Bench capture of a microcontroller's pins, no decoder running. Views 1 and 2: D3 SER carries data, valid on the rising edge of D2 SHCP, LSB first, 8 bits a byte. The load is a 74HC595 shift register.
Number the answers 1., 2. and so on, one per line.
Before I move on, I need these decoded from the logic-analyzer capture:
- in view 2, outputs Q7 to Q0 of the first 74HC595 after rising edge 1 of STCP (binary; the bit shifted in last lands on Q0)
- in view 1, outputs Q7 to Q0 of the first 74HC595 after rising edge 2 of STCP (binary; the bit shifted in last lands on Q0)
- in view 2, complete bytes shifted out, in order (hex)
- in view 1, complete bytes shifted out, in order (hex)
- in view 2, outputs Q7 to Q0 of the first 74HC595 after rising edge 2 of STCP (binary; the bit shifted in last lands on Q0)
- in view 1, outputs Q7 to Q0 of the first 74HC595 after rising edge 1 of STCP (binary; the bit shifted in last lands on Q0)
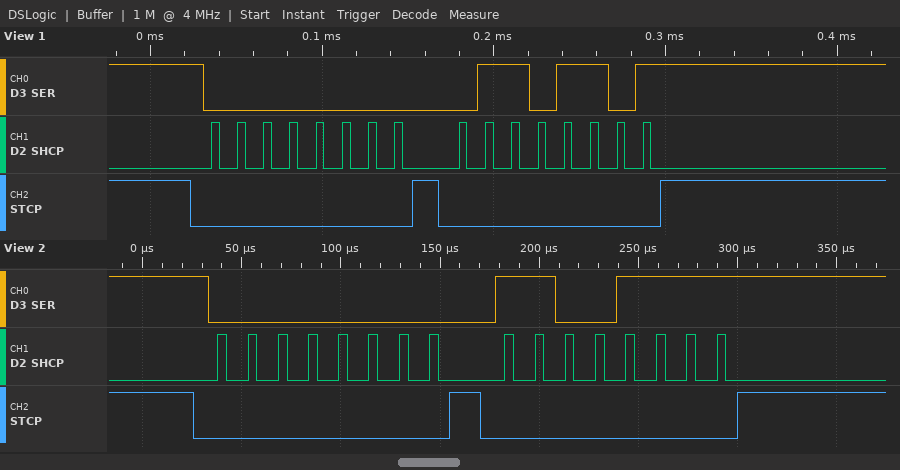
1. 00000000
2. 01101101
3. 00 F3
4. 00 B6
5. 11001111
6. 00000000
